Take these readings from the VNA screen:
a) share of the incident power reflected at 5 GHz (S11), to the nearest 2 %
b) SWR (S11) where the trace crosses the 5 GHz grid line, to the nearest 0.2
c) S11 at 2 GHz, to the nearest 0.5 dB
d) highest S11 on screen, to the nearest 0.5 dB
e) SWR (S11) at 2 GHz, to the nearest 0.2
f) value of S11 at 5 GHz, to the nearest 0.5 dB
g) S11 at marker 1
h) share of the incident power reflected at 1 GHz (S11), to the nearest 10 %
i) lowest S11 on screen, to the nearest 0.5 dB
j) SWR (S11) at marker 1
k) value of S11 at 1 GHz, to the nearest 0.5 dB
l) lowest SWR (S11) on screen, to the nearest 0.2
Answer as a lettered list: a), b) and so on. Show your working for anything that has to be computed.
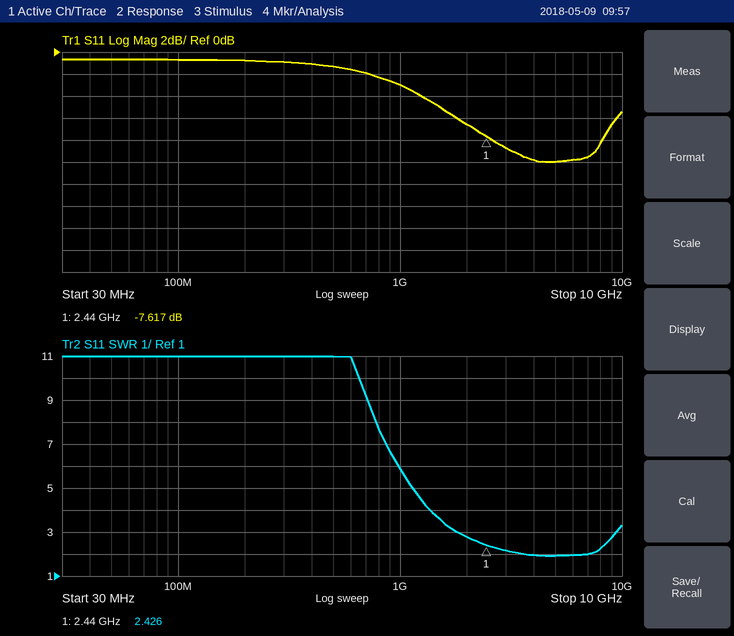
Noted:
a) 10^(-10/10) ≈ 10 %
b) 2.0
c) -6.5 dB
d) -0.5 dB
e) 2.8
f) -10.0 dB
g) -7.617 dB
h) 10^(-3/10) ≈ 50 %
i) -10.0 dB
j) 2.426
k) -3.0 dB
l) 2.0
